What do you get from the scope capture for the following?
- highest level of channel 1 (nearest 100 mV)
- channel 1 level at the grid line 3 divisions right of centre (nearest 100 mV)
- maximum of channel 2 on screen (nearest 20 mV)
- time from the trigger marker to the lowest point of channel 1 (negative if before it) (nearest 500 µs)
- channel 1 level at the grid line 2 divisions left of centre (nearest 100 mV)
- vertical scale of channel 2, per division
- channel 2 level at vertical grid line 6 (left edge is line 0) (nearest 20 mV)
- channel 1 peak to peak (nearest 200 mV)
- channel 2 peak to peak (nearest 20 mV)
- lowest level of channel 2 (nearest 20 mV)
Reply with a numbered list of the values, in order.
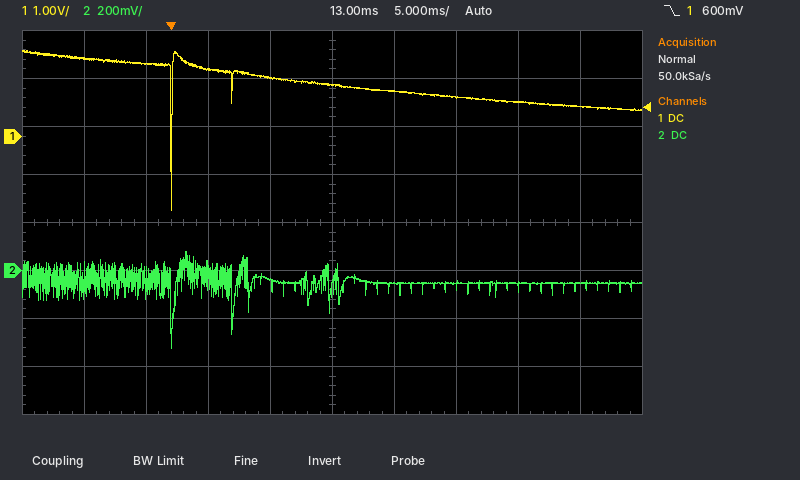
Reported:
1. 1.8 V
2. 700 mV
3. 80 mV
4. 0.0 ms
5. 1.4 V
6. 200 mV
7. -60 mV
8. 3.4 V
9. 400 mV
10. -320 mV
